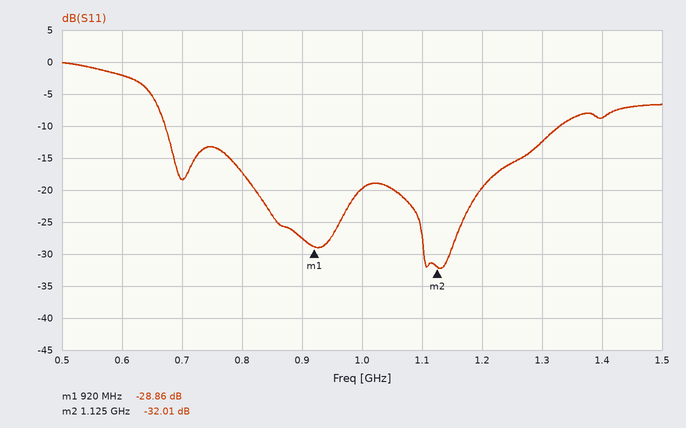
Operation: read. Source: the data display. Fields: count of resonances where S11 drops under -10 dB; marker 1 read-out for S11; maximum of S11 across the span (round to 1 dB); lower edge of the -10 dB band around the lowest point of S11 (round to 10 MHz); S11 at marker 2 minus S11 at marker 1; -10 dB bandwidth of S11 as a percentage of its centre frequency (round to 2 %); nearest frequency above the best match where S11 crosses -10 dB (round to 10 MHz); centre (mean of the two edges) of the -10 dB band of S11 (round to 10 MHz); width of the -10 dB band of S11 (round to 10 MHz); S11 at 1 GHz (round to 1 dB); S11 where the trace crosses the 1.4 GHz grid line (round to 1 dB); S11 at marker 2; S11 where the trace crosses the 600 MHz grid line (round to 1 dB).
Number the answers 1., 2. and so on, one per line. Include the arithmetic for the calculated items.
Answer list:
1. 3
2. -28.86 dB
3. 0 dB
4. 670 MHz
5. -32.01 − (-28.86) = -3.15 dB
6. 660 MHz / 1 GHz ≈ 66 %
7. 1.33 GHz
8. 1.00 GHz
9. 1.33 GHz − 670 MHz = 660 MHz
10. -20 dB
11. -9 dB
12. -32.01 dB
13. -2 dB
